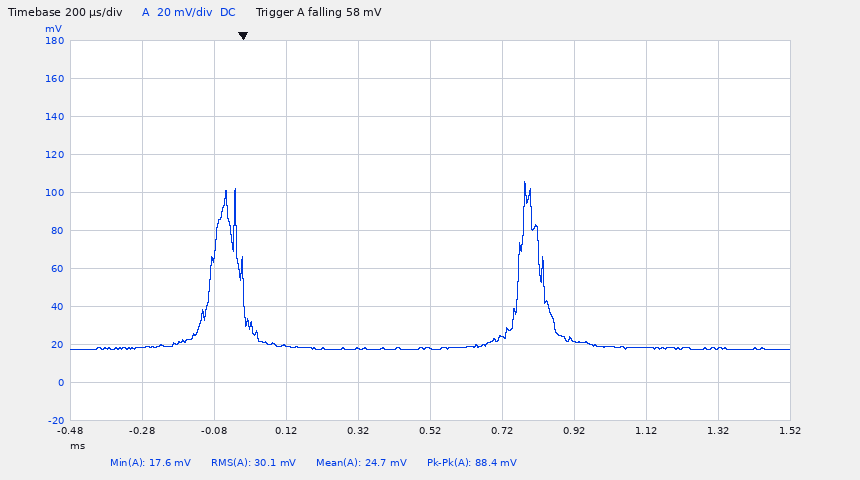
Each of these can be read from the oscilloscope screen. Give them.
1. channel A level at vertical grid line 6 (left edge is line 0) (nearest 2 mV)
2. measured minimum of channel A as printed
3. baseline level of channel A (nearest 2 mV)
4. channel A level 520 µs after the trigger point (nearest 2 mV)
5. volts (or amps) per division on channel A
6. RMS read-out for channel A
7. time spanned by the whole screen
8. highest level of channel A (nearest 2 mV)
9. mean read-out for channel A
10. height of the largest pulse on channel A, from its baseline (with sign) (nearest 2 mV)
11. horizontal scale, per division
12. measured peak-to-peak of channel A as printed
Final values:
24 mV
17.6 mV
18 mV
18 mV
20 mV
30.1 mV
2 ms
106 mV
24.7 mV
+88 mV
200 µs
88.4 mV
